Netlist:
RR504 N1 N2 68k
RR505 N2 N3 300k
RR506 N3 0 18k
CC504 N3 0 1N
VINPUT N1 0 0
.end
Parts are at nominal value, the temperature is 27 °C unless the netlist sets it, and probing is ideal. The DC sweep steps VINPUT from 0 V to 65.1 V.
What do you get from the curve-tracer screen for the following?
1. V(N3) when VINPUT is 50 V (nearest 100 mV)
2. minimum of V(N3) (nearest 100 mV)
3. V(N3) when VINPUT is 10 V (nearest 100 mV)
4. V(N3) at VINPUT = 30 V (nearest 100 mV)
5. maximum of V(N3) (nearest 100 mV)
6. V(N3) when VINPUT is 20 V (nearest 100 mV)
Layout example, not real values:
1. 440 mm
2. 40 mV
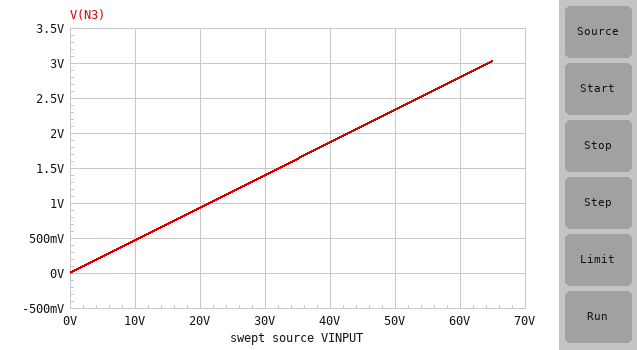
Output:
1. 2.3 V
2. 0 V
3. 500 mV
4. 1.4 V
5. 3.0 V
6. 900 mV
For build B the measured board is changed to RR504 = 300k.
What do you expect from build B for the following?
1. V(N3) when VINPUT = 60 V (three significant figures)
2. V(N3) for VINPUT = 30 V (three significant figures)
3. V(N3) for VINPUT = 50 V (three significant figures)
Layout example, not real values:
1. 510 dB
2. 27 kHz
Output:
1. 1.75 V
2. 874 mV
3. 1.46 V
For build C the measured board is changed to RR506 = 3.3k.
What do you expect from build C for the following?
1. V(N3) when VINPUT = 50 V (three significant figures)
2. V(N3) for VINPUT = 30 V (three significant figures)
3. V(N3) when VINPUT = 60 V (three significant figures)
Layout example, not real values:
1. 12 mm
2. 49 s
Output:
1. 444 mV
2. 267 mV
3. 533 mV
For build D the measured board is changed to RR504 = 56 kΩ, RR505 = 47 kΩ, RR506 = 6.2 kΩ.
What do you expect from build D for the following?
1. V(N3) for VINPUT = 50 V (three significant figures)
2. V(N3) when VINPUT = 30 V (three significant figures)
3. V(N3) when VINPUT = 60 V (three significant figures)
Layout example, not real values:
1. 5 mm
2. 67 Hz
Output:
1. 2.84 V
2. 1.70 V
3. 3.41 V
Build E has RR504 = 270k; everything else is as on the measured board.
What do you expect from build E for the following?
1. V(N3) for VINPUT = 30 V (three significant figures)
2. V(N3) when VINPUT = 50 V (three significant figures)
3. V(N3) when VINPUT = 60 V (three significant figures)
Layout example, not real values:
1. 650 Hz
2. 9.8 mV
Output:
1. 918 mV
2. 1.53 V
3. 1.84 V
